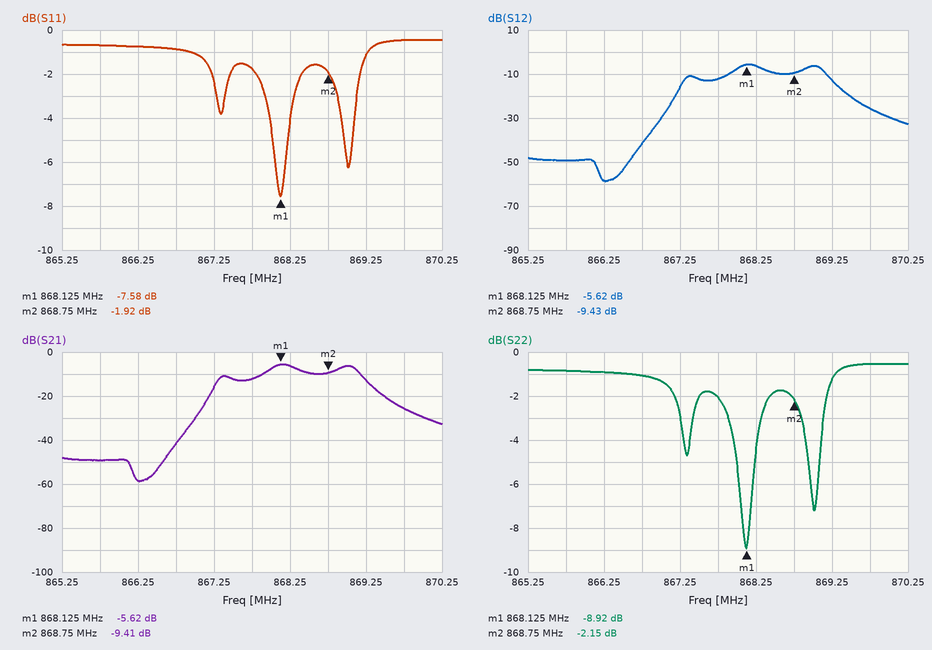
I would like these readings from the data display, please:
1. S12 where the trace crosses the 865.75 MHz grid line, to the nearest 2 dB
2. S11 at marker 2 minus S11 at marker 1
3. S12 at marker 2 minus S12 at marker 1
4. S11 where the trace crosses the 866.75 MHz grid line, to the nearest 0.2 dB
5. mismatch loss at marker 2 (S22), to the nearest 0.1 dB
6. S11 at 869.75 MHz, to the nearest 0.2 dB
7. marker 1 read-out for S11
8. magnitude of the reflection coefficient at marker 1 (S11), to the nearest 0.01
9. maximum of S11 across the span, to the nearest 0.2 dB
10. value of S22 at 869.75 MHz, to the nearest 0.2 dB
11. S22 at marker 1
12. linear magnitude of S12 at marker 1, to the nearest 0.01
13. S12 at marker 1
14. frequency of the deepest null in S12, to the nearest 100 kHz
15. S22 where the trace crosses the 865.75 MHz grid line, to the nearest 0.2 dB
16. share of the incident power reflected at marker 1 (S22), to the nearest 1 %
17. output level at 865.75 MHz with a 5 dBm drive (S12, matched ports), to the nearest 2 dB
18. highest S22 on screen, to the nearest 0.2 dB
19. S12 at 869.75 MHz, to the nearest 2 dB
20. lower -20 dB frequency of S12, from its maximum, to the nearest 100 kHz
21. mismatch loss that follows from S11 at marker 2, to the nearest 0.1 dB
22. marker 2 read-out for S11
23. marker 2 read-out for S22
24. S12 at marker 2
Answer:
-50 dB
5.66 dB
-3.81 dB
-0.8 dB
4.1 dB
-0.4 dB
-7.58 dB
0.42
-0.4 dB
-0.6 dB
-8.92 dB
0.52
-5.62 dB
866.3 MHz
-0.8 dB
13 %
-44 dBm
-0.6 dB
-26 dB
867.1 MHz
4.5 dB
-1.92 dB
-2.15 dB
-9.43 dB
